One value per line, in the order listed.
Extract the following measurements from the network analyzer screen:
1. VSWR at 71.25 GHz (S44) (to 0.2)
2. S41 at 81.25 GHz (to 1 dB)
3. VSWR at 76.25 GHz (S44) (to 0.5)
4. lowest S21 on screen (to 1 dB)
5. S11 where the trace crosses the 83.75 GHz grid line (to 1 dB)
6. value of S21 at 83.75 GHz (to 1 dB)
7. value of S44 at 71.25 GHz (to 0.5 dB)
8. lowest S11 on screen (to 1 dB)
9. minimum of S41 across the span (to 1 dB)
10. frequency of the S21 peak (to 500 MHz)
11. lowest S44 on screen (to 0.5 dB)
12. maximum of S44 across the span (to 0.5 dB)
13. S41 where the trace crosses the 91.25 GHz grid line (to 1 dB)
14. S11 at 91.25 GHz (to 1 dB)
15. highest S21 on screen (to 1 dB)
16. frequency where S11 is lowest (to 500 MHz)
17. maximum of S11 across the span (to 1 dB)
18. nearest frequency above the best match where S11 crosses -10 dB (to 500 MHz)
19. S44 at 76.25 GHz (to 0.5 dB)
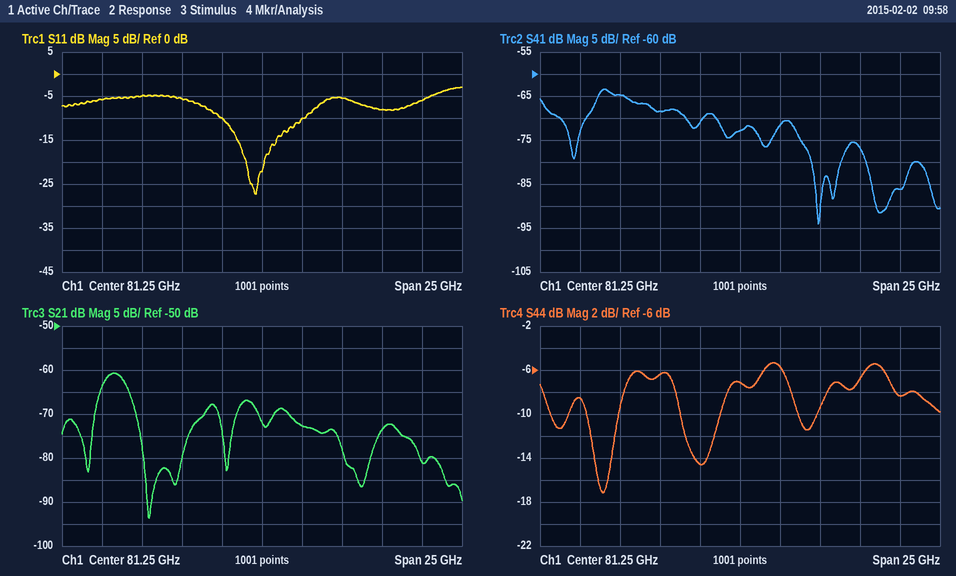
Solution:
2.2
-73 dB
3.0
-94 dB
-10 dB
-73 dB
-8.5 dB
-27 dB
-94 dB
72.0 GHz
-17.0 dB
-5.5 dB
-86 dB
-6 dB
-61 dB
81.0 GHz
-3 dB
84.0 GHz
-6.5 dB
